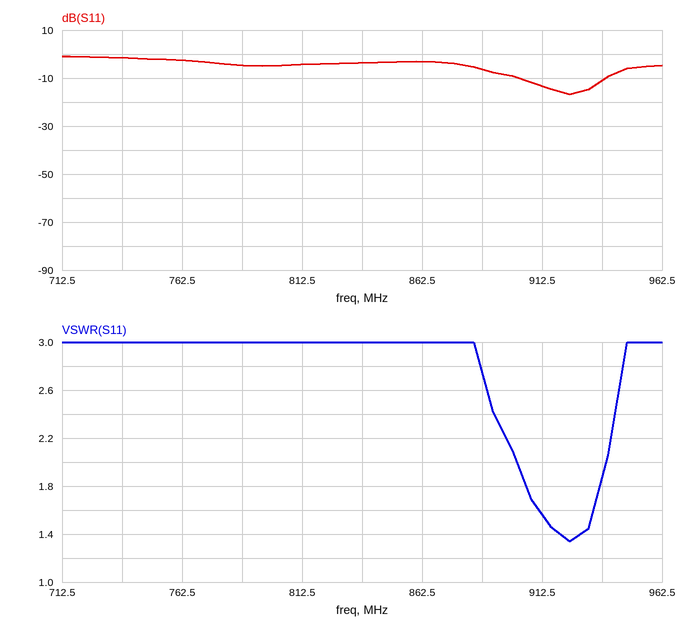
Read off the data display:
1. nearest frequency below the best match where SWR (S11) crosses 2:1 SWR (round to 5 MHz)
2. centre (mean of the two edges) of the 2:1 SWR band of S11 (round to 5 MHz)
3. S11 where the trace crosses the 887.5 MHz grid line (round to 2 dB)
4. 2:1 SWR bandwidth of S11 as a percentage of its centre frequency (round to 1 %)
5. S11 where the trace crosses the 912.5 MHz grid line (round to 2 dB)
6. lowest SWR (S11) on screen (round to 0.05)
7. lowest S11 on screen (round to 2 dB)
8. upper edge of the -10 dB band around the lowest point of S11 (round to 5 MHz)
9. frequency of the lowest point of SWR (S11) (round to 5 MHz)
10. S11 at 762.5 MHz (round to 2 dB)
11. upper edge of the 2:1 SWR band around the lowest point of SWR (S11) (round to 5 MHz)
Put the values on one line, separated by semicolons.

900 MHz; 920 MHz; -6 dB; 4 %; -14 dB; 1.35; -16 dB; 940 MHz; 925 MHz; -2 dB; 940 MHz
